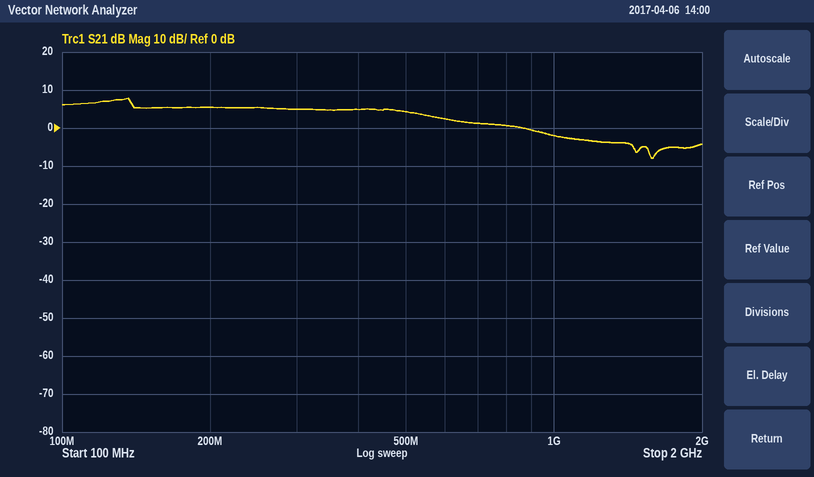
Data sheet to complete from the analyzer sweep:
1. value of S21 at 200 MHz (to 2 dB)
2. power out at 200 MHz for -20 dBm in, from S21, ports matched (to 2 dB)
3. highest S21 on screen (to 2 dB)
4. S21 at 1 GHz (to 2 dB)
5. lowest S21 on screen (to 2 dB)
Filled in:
6 dB
-14 dBm
8 dB
-2 dB
-8 dB
